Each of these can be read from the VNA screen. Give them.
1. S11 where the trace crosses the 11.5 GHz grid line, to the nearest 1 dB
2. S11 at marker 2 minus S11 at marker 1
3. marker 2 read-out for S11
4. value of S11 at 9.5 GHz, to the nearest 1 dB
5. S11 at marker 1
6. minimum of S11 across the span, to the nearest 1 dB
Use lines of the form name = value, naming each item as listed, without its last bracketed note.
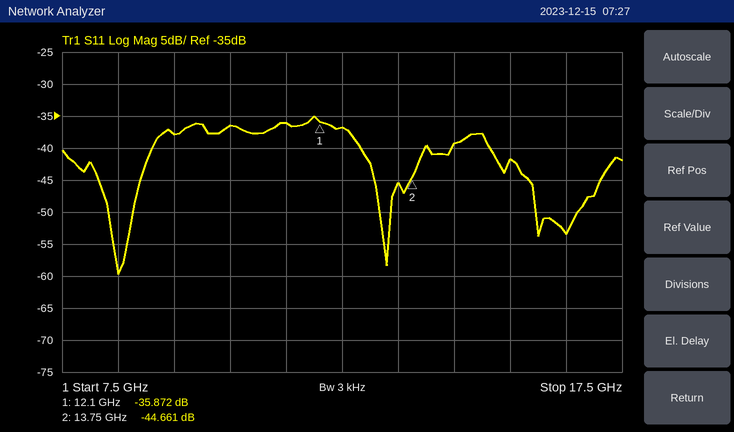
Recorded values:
S11 where the trace crosses the 11.5 GHz grid line, to the nearest 1 dB = -36 dB
S11 at marker 2 minus S11 at marker 1 = -8.789 dB
marker 2 read-out for S11 = -44.661 dB
value of S11 at 9.5 GHz, to the nearest 1 dB = -38 dB
S11 at marker 1 = -35.872 dB
minimum of S11 across the span, to the nearest 1 dB = -60 dB
